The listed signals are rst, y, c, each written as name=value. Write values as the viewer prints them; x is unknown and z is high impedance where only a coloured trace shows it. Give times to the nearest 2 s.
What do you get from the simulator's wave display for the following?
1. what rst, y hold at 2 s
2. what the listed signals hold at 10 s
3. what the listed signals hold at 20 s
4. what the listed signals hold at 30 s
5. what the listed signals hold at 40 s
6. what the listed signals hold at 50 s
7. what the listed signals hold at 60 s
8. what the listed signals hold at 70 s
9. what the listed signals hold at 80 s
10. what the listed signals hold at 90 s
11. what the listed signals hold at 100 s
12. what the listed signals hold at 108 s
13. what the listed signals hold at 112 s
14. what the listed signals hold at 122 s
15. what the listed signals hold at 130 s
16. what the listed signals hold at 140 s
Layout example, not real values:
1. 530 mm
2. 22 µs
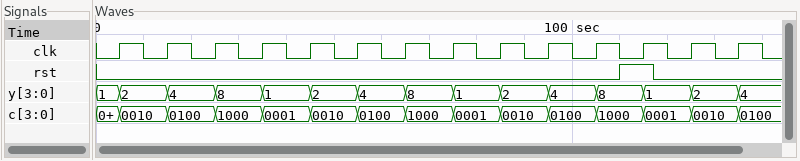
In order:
1. rst=0, y=1
2. rst=0, y=2, c=0010
3. rst=0, y=4, c=0100
4. rst=0, y=8, c=1000
5. rst=0, y=1, c=0001
6. rst=0, y=2, c=0010
7. rst=0, y=4, c=0100
8. rst=0, y=8, c=1000
9. rst=0, y=1, c=0001
10. rst=0, y=2, c=0010
11. rst=0, y=4, c=0100
12. rst=0, y=8, c=1000
13. rst=1, y=8, c=1000
14. rst=0, y=1, c=0001
15. rst=0, y=2, c=0010
16. rst=0, y=4, c=0100
